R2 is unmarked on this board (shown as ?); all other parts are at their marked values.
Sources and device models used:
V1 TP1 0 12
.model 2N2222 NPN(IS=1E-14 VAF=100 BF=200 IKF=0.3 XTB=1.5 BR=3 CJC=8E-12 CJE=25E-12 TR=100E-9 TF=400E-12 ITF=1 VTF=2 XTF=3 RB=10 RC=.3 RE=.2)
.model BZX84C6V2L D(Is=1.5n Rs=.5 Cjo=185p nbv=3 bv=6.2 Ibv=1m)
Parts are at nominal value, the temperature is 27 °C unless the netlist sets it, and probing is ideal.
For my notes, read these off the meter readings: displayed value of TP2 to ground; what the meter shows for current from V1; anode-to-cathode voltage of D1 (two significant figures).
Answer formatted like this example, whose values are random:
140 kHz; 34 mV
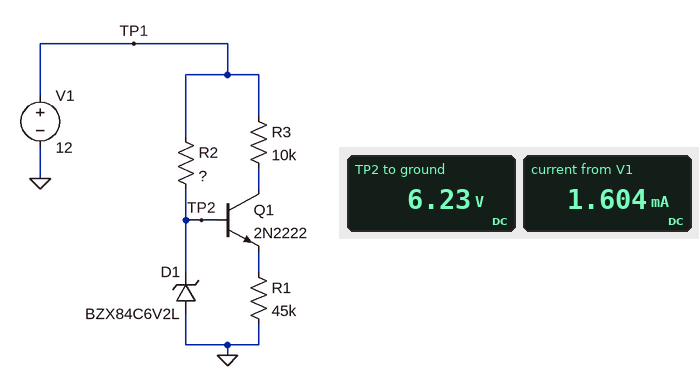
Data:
6.23 V; 1.604 mA; -6.2 V
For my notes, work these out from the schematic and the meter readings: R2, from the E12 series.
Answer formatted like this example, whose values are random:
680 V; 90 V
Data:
3.9 kΩ
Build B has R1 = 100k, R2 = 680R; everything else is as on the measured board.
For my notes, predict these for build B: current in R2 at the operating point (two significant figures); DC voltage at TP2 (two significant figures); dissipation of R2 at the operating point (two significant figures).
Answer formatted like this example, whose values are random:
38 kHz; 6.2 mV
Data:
8.3 mA; 6.4 V; 47 mW
